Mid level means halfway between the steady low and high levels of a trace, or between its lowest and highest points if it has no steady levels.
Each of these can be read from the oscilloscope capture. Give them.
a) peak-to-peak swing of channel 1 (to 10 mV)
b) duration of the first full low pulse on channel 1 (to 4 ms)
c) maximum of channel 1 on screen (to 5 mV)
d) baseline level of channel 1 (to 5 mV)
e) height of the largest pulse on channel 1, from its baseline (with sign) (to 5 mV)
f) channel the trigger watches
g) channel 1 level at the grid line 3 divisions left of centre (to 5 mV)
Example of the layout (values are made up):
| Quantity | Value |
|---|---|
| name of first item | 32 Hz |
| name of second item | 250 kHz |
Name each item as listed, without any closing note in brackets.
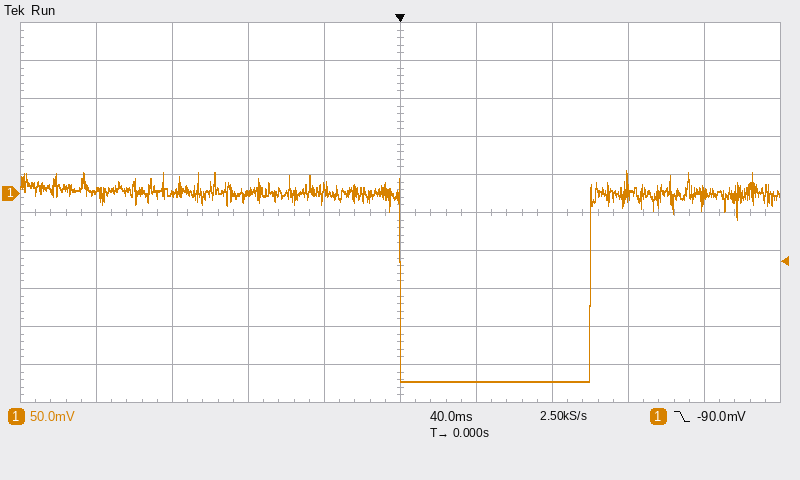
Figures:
| Quantity | Value |
|---|---|
| peak-to-peak swing of channel 1 | 280 mV |
| duration of the first full low pulse on channel 1 | 100 ms |
| maximum of channel 1 on screen | 30 mV |
| baseline level of channel 1 | 0 mV |
| height of the largest pulse on channel 1, from its baseline (with sign) | -250 mV |
| channel the trigger watches | channel 1 |
| channel 1 level at the grid line 3 divisions left of centre | 0 mV |
